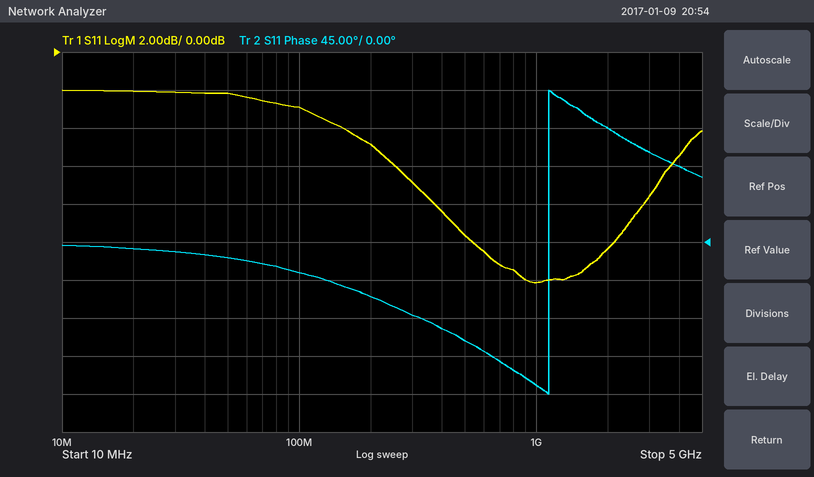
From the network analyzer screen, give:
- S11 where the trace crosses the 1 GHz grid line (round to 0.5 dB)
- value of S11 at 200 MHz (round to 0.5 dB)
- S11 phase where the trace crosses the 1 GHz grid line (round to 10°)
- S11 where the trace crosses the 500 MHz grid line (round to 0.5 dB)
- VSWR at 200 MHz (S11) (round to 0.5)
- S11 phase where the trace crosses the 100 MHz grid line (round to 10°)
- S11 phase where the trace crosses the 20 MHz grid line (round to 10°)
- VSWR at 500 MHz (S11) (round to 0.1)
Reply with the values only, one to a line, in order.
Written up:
-12.0 dB
-5.0 dB
-170°
-9.5 dB
3.5
-40°
-10°
2.0
